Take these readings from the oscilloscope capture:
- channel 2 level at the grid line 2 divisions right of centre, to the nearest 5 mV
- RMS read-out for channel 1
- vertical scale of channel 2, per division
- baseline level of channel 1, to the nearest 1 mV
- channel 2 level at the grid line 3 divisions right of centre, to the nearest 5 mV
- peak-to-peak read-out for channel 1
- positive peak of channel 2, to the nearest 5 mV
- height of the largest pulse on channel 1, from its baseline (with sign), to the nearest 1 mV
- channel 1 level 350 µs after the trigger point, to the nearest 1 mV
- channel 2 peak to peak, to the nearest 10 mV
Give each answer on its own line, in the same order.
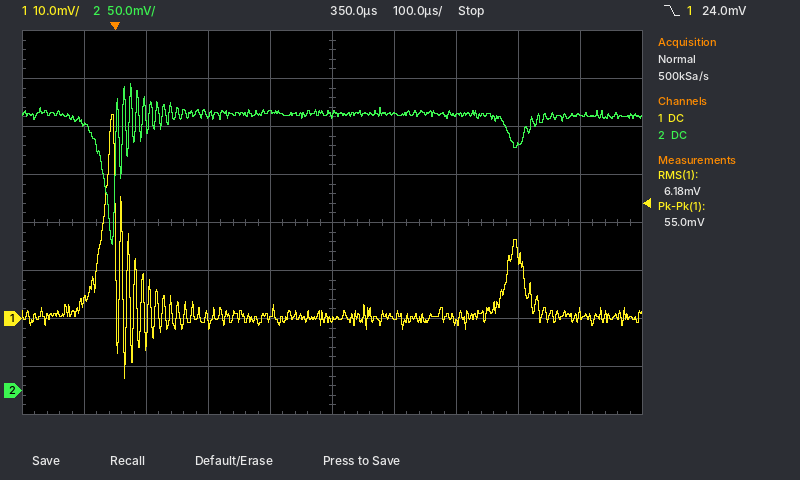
285 mV
6.18 mV
50 mV
0 mV
255 mV
55.0 mV
320 mV
+42 mV
0 mV
170 mV
